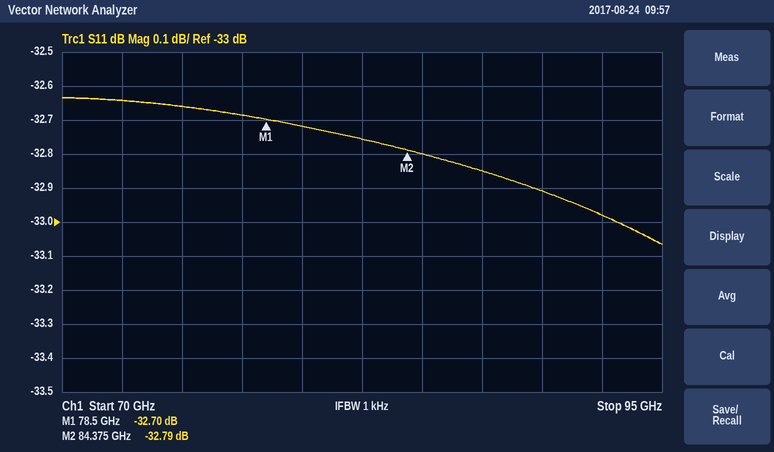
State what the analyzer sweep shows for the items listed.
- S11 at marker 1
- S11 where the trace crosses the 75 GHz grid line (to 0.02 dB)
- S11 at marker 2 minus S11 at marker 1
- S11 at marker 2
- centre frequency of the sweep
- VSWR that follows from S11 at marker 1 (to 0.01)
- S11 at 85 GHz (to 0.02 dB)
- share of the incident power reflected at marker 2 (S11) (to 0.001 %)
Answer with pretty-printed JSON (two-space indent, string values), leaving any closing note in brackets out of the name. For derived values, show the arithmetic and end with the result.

{
  "S11 at marker 1": "-32.70 dB",
  "S11 where the trace crosses the 75 GHz grid line": "-32.66 dB",
  "S11 at marker 2 minus S11 at marker 1": "-32.79 − (-32.7) = -0.09 dB",
  "S11 at marker 2": "-32.79 dB",
  "centre frequency of the sweep": "82.5 GHz",
  "VSWR that follows from S11 at marker 1": "(1 + 0.0232)/(1 − 0.0232) ≈ 1.05",
  "S11 at 85 GHz": "-32.80 dB",
  "share of the incident power reflected at marker 2 (S11)": "10^(-32.79/10) ≈ 0.053 %"
}
